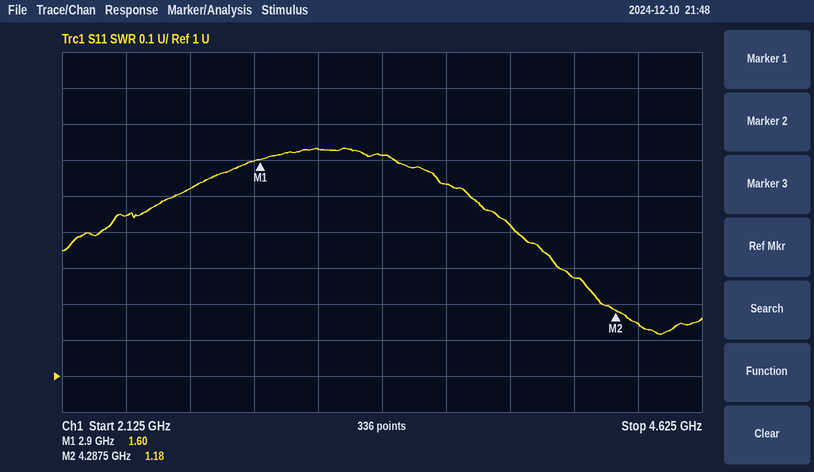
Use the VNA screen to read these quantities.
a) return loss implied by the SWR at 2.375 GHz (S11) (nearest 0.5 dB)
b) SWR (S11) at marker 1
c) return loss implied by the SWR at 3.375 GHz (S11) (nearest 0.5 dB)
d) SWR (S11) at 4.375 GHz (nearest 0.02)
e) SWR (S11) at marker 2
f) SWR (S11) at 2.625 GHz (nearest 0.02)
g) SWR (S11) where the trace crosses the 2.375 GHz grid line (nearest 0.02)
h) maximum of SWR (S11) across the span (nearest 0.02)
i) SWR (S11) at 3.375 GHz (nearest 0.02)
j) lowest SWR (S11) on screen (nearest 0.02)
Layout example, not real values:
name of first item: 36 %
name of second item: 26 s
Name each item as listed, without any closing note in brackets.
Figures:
return loss implied by the SWR at 2.375 GHz (S11): 15.0 dB
SWR (S11) at marker 1: 1.60
return loss implied by the SWR at 3.375 GHz (S11): 12.5 dB
SWR (S11) at 4.375 GHz: 1.14
SWR (S11) at marker 2: 1.18
SWR (S11) at 2.625 GHz: 1.52
SWR (S11) where the trace crosses the 2.375 GHz grid line: 1.44
maximum of SWR (S11) across the span: 1.64
SWR (S11) at 3.375 GHz: 1.62
lowest SWR (S11) on screen: 1.12
